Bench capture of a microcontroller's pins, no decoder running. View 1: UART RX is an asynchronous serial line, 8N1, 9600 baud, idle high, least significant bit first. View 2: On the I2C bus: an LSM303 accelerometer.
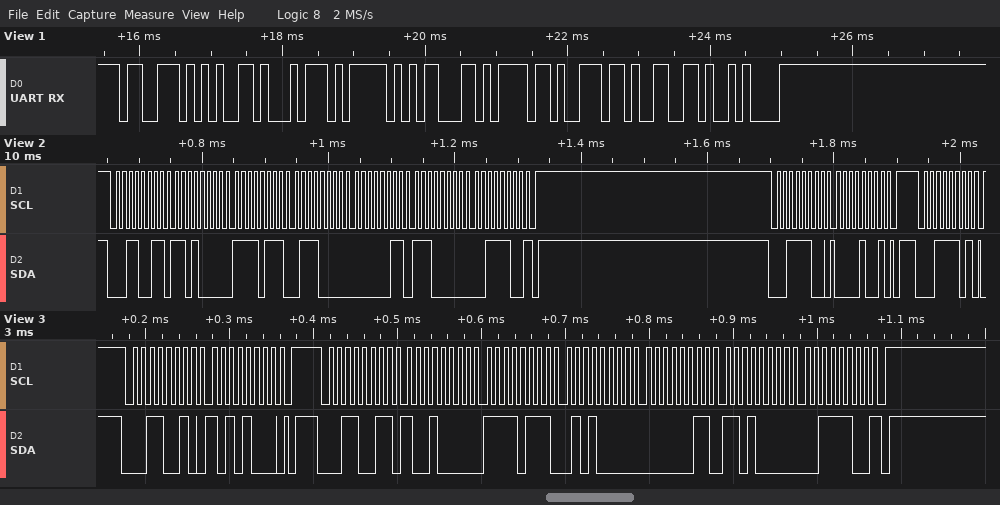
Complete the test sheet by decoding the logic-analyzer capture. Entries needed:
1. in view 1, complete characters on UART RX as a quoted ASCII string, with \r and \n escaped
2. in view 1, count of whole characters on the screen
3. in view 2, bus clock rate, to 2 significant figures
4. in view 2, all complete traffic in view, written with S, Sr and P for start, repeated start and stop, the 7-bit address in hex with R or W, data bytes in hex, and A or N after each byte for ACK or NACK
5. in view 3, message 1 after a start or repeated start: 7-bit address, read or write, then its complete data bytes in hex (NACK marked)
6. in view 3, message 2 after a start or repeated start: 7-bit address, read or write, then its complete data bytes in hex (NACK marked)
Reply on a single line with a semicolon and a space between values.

"set_conf\n"; 9; 100 kHz; S 19R A D0 A F7 A 70 A 03 A E0 A 3C N P S 1EW A 09 A P S 1ER A; 0x19 write: A8; 0x19 read: 90 F7 50 03 D0 3C NACK
